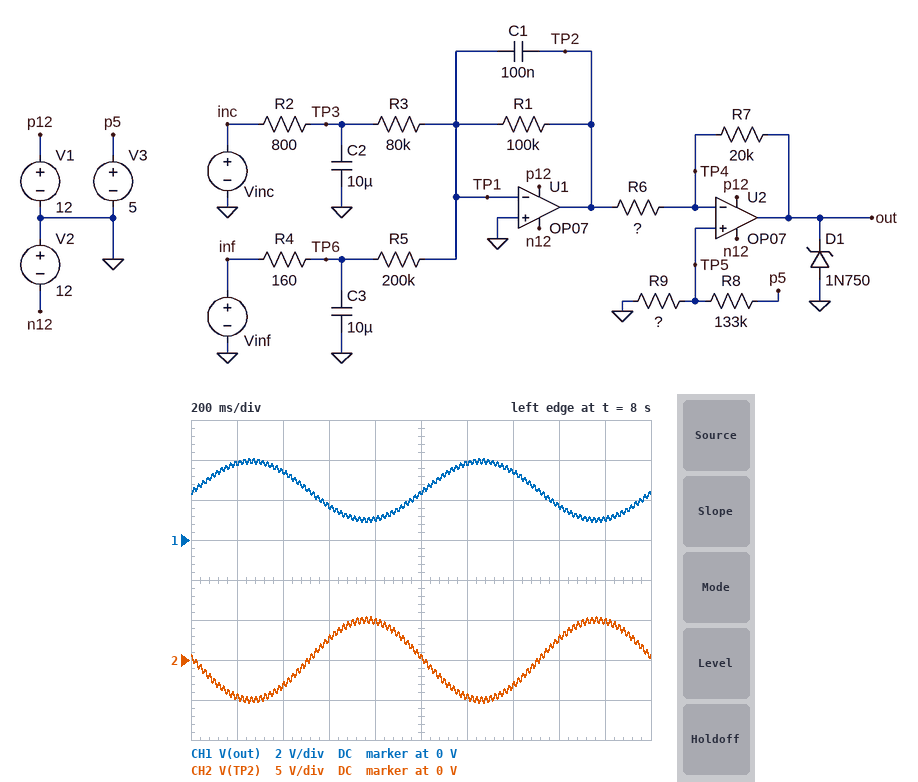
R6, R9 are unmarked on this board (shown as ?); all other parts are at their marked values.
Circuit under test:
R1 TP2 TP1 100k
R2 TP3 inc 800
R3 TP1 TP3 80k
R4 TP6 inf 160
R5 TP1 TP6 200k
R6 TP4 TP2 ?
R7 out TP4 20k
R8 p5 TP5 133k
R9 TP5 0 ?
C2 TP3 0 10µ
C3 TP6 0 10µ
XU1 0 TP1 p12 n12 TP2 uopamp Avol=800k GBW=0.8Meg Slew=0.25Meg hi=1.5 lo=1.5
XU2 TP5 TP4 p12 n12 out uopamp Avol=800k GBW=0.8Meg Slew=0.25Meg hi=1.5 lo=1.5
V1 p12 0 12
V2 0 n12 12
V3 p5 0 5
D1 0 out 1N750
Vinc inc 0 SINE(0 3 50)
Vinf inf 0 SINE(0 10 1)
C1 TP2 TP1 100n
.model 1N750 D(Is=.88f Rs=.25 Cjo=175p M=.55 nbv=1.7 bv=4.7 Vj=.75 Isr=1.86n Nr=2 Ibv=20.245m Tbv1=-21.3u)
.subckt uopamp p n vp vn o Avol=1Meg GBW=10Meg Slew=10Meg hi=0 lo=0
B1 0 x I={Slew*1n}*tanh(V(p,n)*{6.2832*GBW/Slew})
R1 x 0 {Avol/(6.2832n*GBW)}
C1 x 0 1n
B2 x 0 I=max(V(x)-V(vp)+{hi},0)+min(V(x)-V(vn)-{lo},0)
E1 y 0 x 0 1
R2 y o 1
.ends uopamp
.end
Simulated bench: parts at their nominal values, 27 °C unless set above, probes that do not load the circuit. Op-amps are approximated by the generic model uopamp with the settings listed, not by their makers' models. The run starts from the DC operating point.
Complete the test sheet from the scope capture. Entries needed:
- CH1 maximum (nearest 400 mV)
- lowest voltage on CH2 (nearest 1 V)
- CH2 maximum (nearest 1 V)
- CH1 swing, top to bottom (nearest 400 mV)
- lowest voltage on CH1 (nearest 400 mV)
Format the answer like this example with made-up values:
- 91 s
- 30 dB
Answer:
- 4.0 V
- -5 V
- 5 V
- 3.2 V
- 800 mV
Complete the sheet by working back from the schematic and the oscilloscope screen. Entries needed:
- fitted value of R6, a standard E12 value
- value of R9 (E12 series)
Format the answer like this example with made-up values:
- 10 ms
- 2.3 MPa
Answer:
- 68 kΩ
- 82 kΩ
